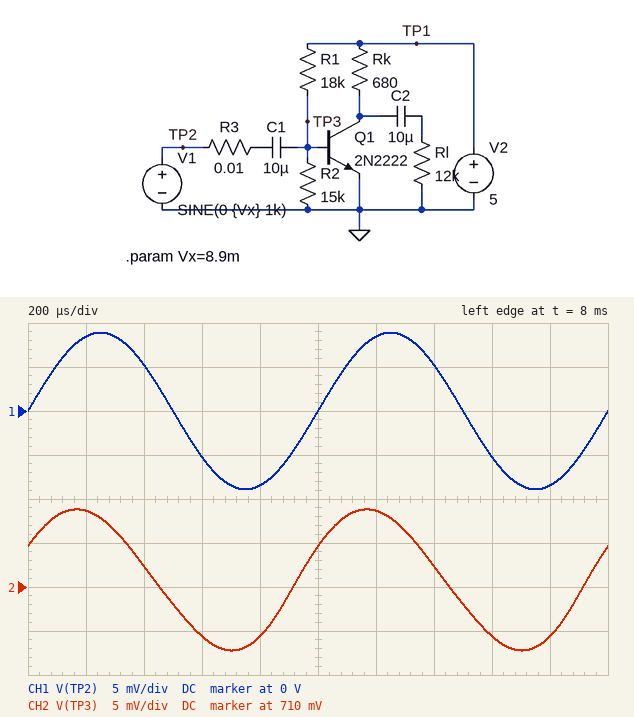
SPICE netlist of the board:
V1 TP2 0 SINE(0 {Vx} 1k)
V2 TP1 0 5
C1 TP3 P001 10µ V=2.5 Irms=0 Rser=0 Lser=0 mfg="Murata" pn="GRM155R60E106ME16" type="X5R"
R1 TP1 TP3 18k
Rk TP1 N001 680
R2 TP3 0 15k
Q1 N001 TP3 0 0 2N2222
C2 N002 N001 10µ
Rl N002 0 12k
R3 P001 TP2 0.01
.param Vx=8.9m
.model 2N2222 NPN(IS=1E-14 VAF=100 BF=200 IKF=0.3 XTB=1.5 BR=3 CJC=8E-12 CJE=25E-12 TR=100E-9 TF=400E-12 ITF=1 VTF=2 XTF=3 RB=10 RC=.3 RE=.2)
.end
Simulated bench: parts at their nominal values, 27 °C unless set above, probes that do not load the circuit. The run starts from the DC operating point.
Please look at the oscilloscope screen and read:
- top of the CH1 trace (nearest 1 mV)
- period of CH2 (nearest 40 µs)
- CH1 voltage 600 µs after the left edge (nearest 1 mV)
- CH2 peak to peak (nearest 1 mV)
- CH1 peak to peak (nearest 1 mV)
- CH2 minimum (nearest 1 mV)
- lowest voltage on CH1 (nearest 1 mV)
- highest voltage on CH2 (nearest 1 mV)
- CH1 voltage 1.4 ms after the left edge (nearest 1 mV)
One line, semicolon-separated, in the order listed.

9 mV; 1.00 ms; -5 mV; 16 mV; 18 mV; 703 mV; -9 mV; 719 mV; 5 mV
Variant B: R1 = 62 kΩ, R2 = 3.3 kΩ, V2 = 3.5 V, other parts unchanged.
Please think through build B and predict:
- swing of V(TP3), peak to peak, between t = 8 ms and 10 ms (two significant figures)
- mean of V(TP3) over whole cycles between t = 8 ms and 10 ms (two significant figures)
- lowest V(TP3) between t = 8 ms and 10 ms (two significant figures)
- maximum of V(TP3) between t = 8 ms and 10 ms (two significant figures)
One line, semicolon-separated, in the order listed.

18 mV; 180 mV; 170 mV; 190 mV
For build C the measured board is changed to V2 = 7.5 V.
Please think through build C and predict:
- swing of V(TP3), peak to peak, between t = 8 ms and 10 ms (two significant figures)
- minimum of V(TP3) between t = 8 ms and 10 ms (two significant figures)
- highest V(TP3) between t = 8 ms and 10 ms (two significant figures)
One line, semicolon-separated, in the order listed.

14 mV; 720 mV; 730 mV
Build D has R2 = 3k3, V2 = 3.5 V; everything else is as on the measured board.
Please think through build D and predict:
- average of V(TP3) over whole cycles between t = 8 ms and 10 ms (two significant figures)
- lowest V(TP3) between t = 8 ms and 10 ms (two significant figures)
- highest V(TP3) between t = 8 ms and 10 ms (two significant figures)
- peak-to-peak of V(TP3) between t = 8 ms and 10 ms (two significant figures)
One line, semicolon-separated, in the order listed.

540 mV; 530 mV; 550 mV; 18 mV
